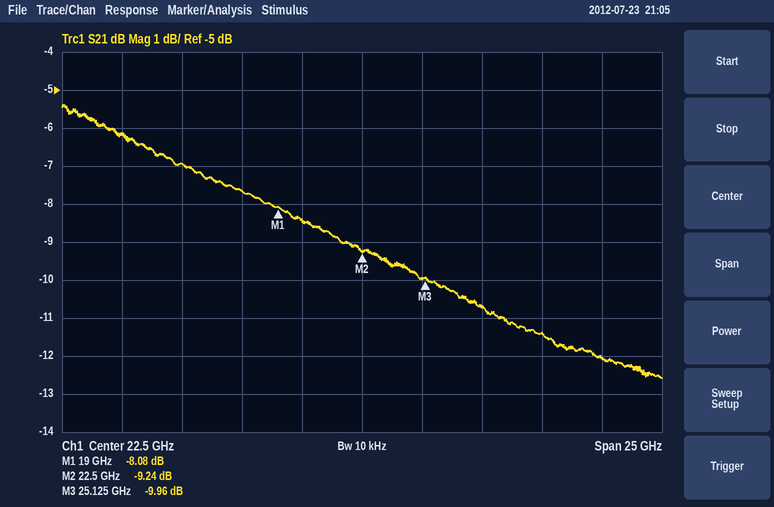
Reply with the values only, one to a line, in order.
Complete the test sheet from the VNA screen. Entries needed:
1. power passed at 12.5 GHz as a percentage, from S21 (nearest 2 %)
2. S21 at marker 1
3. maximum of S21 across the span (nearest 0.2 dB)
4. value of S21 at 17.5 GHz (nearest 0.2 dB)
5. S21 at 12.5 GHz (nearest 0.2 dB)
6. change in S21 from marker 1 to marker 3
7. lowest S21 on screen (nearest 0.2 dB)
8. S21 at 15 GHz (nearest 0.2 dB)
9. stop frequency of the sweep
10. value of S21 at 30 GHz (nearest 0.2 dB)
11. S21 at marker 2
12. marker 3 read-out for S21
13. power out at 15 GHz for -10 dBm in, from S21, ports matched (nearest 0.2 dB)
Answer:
24 %
-8.08 dB
-5.4 dB
-7.6 dB
-6.2 dB
-1.88 dB
-12.6 dB
-7.0 dB
35 GHz
-11.4 dB
-9.24 dB
-9.96 dB
-17.0 dBm
